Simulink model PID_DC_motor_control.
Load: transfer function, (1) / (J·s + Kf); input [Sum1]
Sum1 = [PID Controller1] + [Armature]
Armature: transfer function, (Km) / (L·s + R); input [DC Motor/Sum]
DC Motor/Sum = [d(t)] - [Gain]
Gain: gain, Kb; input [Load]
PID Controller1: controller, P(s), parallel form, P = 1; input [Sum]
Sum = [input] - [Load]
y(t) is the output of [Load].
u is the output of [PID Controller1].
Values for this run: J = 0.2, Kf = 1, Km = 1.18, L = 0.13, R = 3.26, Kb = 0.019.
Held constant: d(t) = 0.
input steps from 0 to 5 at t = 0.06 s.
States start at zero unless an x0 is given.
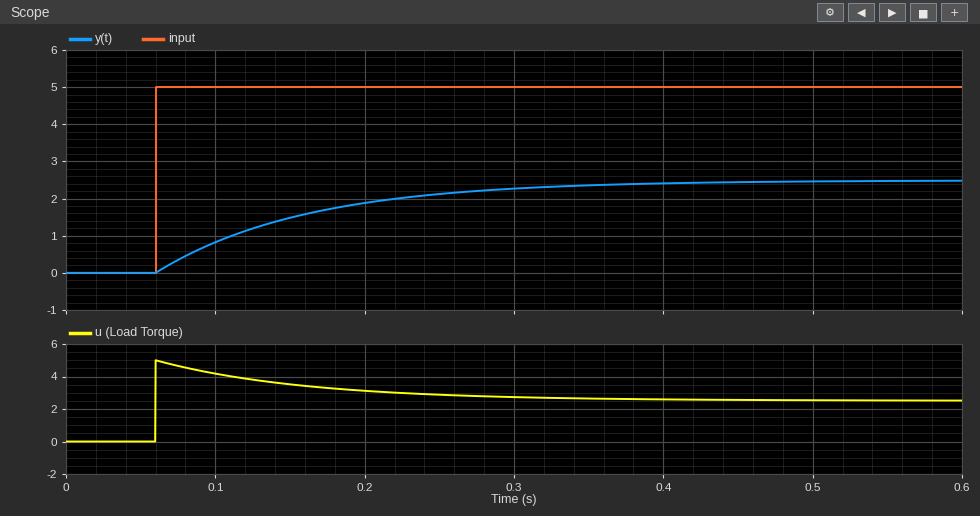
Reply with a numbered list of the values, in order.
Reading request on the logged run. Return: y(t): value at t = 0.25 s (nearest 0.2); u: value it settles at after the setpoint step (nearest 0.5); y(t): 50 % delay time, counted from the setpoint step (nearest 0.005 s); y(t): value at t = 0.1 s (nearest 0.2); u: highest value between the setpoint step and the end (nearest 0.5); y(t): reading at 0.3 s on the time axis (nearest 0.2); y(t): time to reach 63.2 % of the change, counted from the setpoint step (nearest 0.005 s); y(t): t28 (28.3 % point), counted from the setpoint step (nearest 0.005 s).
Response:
1. 2.2
2. 2.5
3. 0.070 s
4. 0.8
5. 5.0
6. 2.2
7. 0.100 s
8. 0.035 s
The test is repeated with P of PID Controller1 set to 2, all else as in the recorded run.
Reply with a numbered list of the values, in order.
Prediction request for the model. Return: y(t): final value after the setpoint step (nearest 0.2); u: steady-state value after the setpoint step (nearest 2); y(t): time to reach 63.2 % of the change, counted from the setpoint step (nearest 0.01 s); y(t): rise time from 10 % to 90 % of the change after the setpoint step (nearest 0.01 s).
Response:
1. 3.4
2. 4
3. 0.07 s
4. 0.15 s
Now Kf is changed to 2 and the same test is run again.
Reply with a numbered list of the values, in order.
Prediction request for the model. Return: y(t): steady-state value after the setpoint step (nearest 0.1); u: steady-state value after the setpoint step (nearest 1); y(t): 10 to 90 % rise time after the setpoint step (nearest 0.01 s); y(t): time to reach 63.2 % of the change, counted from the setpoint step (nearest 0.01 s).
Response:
1. 1.7
2. 3
3. 0.15 s
4. 0.07 s
